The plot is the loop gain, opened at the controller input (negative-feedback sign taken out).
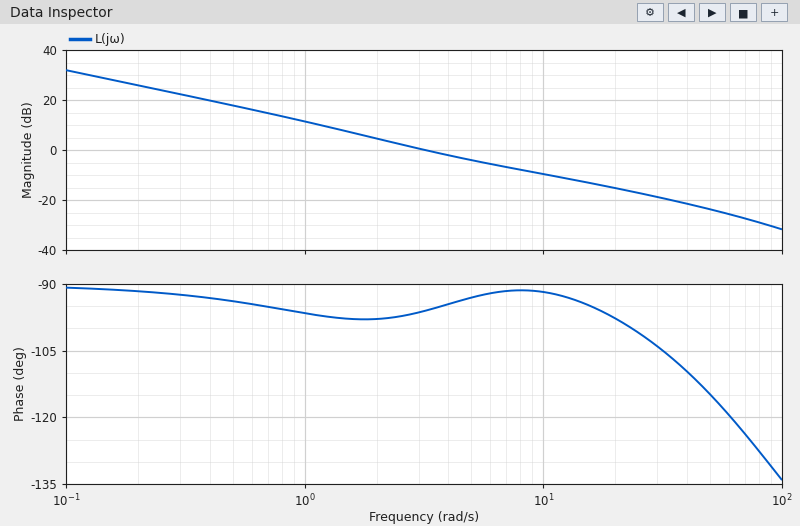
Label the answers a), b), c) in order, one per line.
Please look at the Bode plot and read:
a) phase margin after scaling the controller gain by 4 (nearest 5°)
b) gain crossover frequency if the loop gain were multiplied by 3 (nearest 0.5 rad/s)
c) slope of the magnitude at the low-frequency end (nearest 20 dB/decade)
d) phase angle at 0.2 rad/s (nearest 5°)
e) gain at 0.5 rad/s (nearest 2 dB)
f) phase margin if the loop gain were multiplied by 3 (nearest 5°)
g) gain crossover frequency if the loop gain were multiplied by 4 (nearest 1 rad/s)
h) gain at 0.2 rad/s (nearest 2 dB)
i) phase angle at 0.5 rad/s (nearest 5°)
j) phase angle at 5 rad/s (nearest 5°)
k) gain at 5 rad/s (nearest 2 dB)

a) 85°
b) 10.0 rad/s
c) -20 dB/decade
d) -90°
e) 18 dB
f) 90°
g) 14 rad/s
h) 26 dB
i) -95°
j) -95°
k) -4 dB
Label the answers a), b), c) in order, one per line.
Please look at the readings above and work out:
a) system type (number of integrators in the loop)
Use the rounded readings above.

a) 1
